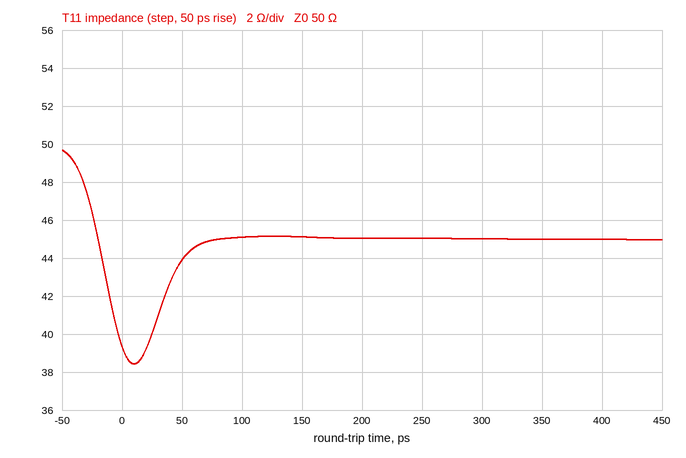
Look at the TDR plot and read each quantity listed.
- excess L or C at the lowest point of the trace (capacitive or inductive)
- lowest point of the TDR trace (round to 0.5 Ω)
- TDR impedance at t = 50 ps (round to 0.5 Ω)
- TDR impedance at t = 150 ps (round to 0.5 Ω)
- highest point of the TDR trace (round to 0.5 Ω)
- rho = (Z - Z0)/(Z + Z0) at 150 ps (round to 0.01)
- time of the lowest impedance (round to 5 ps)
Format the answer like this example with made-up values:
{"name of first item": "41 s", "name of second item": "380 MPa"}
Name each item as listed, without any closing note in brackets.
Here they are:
{"excess L or C at the lowest point of the trace": "capacitive", "lowest point of the TDR trace": "38.5 Ω", "TDR impedance at t = 50 ps": "44.0 Ω", "TDR impedance at t = 150 ps": "45.0 Ω", "highest point of the TDR trace": "49.5 Ω", "rho = (Z - Z0)/(Z + Z0) at 150 ps": "-0.05", "time of the lowest impedance": "10 ps"}
